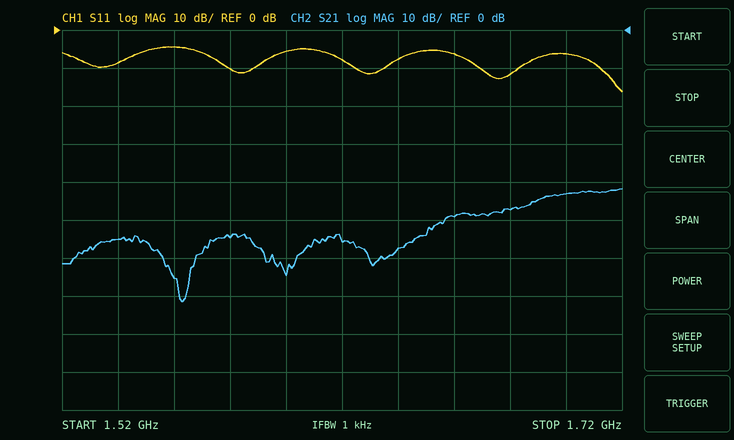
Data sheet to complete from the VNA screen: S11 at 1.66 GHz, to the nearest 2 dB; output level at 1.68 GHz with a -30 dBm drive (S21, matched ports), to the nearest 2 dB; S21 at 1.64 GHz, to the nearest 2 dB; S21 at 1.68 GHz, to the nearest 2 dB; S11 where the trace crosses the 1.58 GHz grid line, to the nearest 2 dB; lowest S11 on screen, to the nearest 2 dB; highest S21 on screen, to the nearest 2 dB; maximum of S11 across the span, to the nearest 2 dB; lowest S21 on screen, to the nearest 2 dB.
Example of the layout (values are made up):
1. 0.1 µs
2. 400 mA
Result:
1. -6 dB
2. -78 dBm
3. -58 dB
4. -48 dB
5. -10 dB
6. -16 dB
7. -42 dB
8. -4 dB
9. -72 dB
